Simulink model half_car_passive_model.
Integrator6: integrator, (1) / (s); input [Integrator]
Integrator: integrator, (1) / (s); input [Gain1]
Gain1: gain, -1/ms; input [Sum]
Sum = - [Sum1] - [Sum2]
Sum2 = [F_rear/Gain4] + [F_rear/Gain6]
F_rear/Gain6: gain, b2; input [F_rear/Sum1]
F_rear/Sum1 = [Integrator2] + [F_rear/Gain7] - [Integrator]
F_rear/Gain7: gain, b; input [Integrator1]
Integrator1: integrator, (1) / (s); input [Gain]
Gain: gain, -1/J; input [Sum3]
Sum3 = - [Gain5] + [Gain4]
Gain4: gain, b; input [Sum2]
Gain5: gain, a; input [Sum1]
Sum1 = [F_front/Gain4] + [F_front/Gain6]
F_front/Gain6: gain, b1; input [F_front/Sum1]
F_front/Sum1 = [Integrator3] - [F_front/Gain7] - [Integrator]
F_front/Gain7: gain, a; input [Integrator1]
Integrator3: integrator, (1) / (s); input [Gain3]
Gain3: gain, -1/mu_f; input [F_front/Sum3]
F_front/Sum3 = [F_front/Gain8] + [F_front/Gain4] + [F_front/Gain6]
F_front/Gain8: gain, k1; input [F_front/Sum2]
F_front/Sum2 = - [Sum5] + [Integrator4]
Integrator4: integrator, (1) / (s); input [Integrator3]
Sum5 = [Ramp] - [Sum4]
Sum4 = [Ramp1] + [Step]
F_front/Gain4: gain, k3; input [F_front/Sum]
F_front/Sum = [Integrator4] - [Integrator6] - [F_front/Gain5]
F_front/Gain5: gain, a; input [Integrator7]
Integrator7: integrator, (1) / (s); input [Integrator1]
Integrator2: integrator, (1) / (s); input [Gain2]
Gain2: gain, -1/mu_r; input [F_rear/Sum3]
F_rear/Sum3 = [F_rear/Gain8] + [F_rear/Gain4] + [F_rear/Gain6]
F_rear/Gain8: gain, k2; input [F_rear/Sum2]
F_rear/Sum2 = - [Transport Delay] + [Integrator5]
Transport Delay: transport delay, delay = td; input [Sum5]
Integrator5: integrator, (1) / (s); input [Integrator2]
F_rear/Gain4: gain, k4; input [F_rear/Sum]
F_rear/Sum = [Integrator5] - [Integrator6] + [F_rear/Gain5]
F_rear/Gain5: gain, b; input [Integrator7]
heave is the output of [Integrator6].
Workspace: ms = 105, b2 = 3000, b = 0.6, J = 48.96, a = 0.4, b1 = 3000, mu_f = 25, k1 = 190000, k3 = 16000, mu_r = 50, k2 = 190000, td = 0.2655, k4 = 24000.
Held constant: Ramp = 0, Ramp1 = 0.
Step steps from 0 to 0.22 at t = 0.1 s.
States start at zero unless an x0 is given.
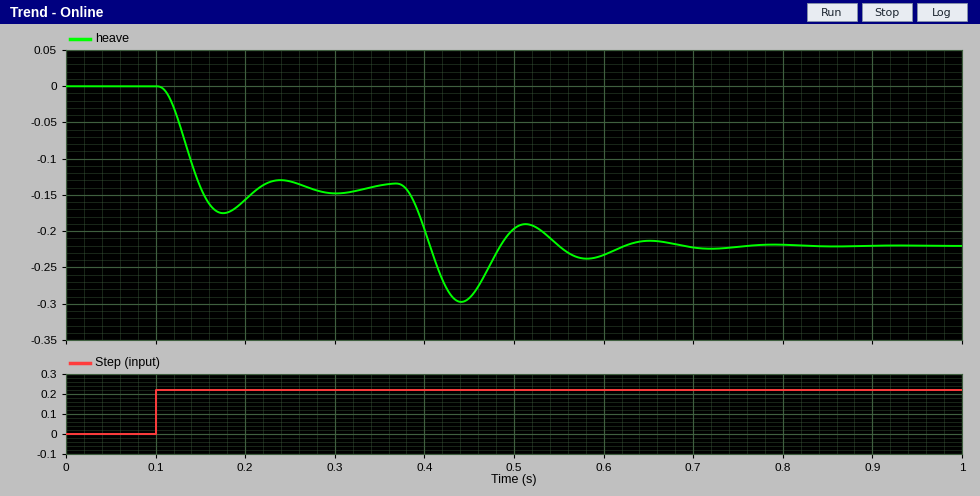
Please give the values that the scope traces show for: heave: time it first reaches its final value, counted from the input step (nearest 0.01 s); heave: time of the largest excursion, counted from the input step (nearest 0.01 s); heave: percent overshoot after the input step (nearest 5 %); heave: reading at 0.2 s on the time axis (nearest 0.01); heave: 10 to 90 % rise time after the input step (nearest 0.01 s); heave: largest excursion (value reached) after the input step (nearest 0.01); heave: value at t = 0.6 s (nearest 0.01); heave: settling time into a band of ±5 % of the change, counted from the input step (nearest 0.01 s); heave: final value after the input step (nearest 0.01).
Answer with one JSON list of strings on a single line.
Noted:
["0.31 s", "0.34 s", "35 %", "-0.16", "0.28 s", "-0.30", "-0.23", "0.50 s", "-0.22"]
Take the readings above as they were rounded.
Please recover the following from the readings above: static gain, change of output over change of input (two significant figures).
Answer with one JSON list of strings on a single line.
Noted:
["-1.0"]
